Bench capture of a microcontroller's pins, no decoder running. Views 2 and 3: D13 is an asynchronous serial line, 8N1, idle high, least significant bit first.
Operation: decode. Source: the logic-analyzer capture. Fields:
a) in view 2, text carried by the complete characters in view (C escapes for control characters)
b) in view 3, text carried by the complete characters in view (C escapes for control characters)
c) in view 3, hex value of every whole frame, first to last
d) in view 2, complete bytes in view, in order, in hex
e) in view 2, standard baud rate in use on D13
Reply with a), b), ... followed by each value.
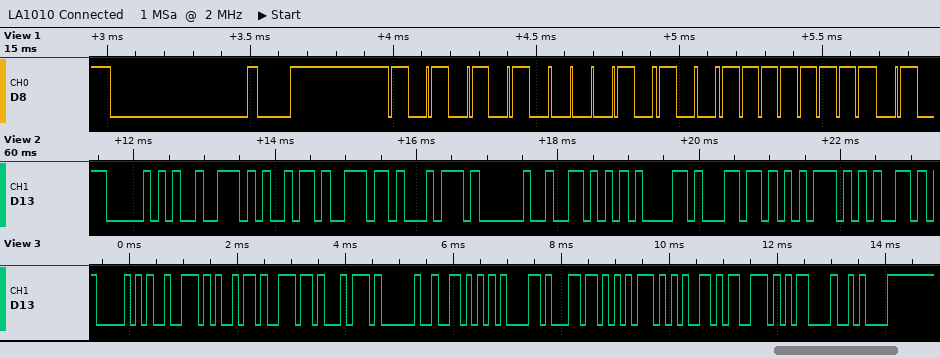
a) "Print Value"
b) "Print Values\r\n"
c) 50 72 69 6E 74 20 56 61 6C 75 65 73 0D 0A
d) 50 72 69 6E 74 20 56 61 6C 75 65
e) 9600 baud
